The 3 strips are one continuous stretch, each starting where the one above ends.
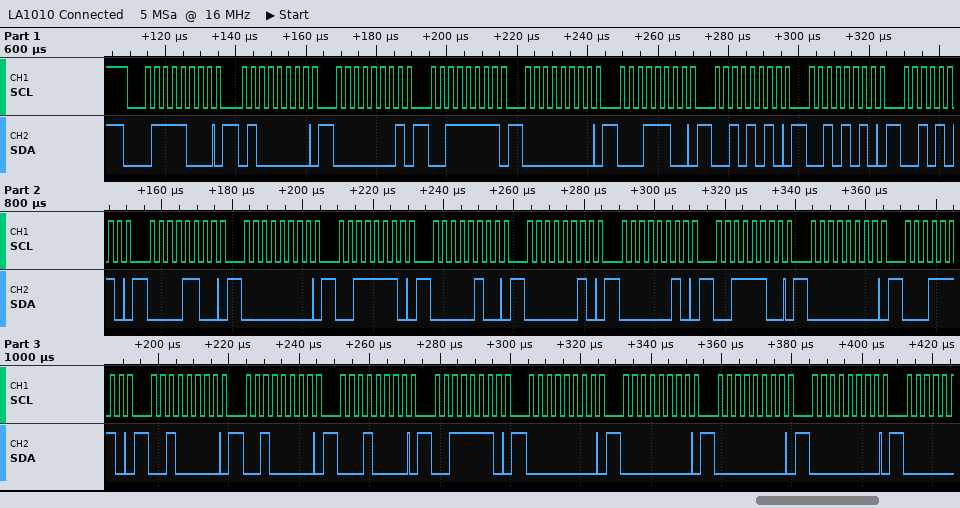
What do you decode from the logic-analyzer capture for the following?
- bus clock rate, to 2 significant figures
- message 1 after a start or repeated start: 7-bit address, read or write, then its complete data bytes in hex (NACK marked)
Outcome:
400 kHz
0x3C write: 40 01 3F 00 1C 2A 2A 2A 0C 00 3E 04 02 02 3C 00 1E 20 20 10 3E 00 00 00 00
